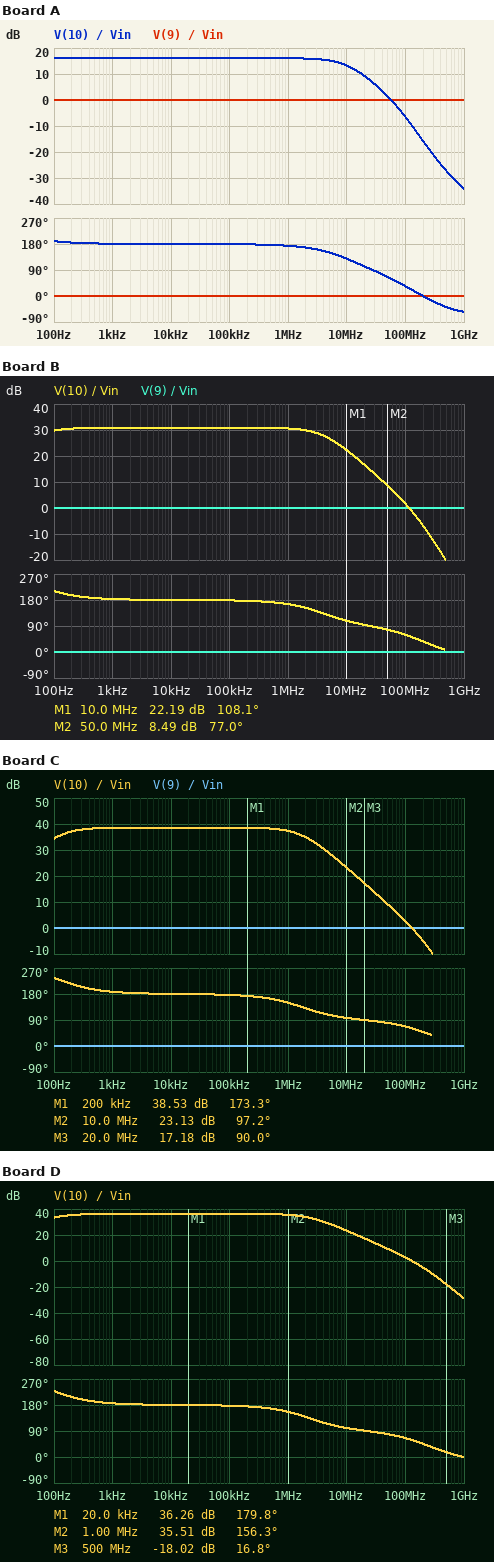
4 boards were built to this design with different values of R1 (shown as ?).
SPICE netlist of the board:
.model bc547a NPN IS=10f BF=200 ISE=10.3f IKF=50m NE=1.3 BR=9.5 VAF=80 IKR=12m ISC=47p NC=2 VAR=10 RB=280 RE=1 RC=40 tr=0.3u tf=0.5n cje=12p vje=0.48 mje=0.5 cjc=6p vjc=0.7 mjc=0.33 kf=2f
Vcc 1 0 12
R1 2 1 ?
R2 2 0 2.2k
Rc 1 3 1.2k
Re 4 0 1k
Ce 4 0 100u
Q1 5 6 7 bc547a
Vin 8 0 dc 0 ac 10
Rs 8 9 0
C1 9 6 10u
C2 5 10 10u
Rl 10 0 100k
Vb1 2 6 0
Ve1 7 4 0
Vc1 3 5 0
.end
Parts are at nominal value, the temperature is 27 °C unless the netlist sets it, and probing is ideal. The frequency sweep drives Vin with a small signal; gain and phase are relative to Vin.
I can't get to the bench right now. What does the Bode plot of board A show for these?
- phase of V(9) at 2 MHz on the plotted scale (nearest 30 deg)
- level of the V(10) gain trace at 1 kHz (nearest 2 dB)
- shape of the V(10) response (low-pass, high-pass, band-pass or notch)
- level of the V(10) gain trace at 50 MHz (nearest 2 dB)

0 deg
16 dB
low-pass
2 dB
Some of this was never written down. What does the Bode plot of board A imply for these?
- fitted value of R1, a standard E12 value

33 kΩ
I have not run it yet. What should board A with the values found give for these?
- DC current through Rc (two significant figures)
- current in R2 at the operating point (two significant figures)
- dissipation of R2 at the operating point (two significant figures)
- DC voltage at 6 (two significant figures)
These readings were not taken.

140 µA
340 µA
250 µW
750 mV
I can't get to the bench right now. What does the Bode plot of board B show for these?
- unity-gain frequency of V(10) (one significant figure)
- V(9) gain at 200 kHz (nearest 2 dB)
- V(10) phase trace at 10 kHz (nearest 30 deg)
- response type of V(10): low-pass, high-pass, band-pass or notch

100 MHz
0 dB
180 deg
low-pass
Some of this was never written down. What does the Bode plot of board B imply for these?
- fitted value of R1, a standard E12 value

15 kΩ
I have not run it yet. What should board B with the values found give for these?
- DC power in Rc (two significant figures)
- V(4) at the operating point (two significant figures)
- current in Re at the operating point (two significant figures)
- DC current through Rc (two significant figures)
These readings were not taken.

890 µW
870 mV
870 µA
860 µA
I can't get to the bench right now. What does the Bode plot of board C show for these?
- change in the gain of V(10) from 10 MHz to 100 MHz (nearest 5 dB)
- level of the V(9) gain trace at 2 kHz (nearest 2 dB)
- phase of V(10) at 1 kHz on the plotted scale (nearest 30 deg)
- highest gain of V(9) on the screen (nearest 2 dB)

-20 dB
0 dB
180 deg
0 dB
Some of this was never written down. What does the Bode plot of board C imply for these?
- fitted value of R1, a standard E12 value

5.6 kΩ
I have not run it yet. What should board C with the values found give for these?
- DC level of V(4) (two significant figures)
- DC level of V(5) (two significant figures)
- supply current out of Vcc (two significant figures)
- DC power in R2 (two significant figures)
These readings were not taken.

2.7 V
8.8 V
4.2 mA
5.1 mW
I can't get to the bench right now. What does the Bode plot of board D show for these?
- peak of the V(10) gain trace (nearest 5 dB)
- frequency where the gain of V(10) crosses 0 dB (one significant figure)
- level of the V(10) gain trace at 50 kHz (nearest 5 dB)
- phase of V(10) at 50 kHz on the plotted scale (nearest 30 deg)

35 dB
100 MHz
35 dB
180 deg
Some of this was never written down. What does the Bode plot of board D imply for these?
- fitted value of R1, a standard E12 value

8.2 kΩ
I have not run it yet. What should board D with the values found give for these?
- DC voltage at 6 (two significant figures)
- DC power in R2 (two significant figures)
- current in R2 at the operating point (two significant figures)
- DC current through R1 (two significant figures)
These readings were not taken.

2.5 V
2.9 mW
1.1 mA
1.2 mA
